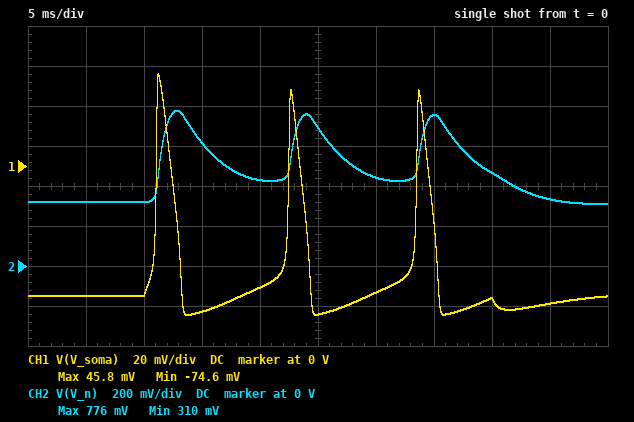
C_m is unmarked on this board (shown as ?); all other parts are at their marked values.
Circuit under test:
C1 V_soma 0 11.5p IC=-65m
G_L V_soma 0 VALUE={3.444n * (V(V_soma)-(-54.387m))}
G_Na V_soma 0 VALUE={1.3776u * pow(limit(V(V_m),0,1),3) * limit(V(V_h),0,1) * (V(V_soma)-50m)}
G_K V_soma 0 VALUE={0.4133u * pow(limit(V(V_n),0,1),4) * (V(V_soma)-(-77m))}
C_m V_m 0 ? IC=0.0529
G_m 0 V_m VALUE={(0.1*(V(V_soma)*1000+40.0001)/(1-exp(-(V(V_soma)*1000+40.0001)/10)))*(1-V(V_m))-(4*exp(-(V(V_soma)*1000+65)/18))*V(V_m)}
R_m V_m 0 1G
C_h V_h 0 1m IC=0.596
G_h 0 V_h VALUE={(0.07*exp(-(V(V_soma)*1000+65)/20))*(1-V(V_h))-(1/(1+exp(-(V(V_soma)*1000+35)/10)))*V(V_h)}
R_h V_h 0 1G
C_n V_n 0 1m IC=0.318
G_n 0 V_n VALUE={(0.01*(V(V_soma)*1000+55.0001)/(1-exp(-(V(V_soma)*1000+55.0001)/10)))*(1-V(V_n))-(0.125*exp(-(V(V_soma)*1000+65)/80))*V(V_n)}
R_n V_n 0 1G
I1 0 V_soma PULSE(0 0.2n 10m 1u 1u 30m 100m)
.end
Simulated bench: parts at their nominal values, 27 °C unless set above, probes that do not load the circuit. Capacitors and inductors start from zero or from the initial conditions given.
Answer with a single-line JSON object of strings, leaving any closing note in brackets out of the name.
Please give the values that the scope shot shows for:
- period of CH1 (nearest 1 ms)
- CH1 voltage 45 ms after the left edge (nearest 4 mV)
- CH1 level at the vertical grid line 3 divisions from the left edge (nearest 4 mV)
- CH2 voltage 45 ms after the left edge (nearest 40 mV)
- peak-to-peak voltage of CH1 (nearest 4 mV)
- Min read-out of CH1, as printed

{"period of CH1": "11 ms", "CH1 voltage 45 ms after the left edge": "-68 mV", "CH1 level at the vertical grid line 3 divisions from the left edge": "-72 mV", "CH2 voltage 45 ms after the left edge": "320 mV", "peak-to-peak voltage of CH1": "120 mV", "Min read-out of CH1, as printed": "-74.6 mV"}
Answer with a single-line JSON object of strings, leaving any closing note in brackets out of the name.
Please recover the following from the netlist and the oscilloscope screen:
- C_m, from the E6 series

{"C_m, from the E6 series": "470 µF"}
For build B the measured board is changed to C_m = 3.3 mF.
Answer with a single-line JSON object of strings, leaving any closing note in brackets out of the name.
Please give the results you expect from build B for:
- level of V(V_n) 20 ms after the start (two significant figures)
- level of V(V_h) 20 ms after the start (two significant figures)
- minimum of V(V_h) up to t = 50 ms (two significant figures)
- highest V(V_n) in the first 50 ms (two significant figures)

{"level of V(V_n) 20 ms after the start": "460 mV", "level of V(V_h) 20 ms after the start": "320 mV", "minimum of V(V_h) up to t = 50 ms": "63 mV", "highest V(V_n) in the first 50 ms": "710 mV"}
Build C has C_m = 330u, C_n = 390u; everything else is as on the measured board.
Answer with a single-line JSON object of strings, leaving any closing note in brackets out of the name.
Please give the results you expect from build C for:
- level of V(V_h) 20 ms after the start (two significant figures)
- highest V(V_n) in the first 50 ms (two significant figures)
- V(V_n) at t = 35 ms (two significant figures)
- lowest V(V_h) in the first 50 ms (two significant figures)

{"level of V(V_h) 20 ms after the start": "180 mV", "highest V(V_n) in the first 50 ms": "860 mV", "V(V_n) at t = 35 ms": "420 mV", "lowest V(V_h) in the first 50 ms": "100 mV"}
